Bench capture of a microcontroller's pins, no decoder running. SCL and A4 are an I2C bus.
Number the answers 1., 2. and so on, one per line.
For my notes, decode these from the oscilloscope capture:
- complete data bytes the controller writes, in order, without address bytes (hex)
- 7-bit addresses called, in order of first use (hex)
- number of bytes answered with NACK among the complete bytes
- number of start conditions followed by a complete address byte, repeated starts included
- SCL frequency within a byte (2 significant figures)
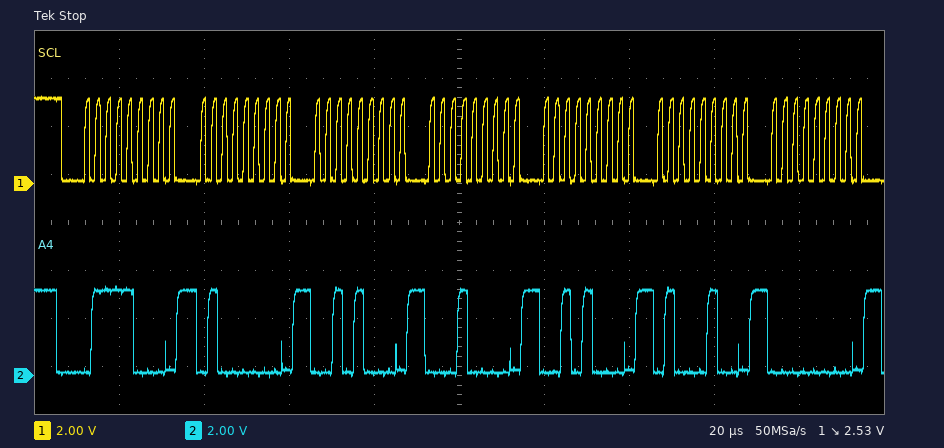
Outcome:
1. 40 28 10 28 44 00
2. 0x3C
3. 0
4. 1
5. 400 kHz
